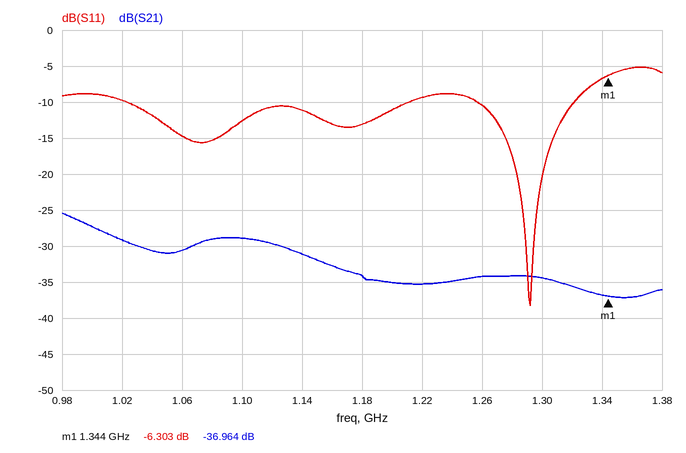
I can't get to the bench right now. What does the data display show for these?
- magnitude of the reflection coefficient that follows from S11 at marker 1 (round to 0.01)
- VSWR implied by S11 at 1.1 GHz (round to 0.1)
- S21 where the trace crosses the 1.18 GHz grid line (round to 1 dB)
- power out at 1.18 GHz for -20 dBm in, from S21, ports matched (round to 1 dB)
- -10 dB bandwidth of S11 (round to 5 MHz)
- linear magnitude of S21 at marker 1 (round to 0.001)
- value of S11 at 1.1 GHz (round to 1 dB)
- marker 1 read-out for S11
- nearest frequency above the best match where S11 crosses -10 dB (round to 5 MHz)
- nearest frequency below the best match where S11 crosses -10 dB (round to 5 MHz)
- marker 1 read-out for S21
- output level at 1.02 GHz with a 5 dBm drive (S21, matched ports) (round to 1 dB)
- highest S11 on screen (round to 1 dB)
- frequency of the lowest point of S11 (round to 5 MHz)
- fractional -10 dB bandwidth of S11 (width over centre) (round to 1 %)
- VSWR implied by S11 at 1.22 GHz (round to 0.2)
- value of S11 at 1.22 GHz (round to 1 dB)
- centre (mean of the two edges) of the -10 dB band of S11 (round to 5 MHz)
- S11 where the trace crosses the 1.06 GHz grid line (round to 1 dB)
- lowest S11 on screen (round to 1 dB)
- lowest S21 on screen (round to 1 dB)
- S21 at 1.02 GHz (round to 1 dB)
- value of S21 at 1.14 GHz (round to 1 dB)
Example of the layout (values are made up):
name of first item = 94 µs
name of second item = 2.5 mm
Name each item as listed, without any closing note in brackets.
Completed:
magnitude of the reflection coefficient that follows from S11 at marker 1 = 0.48
VSWR implied by S11 at 1.1 GHz = 1.6
S21 where the trace crosses the 1.18 GHz grid line = -34 dB
power out at 1.18 GHz for -20 dBm in, from S21, ports matched = -54 dBm
-10 dB bandwidth of S11 = 65 MHz
linear magnitude of S21 at marker 1 = 0.014
value of S11 at 1.1 GHz = -13 dB
marker 1 read-out for S11 = -6.303 dB
nearest frequency above the best match where S11 crosses -10 dB = 1.320 GHz
nearest frequency below the best match where S11 crosses -10 dB = 1.255 GHz
marker 1 read-out for S21 = -36.964 dB
output level at 1.02 GHz with a 5 dBm drive (S21, matched ports) = -24 dBm
highest S11 on screen = -5 dB
frequency of the lowest point of S11 = 1.290 GHz
fractional -10 dB bandwidth of S11 (width over centre) = 5 %
VSWR implied by S11 at 1.22 GHz = 2.0
value of S11 at 1.22 GHz = -9 dB
centre (mean of the two edges) of the -10 dB band of S11 = 1.290 GHz
S11 where the trace crosses the 1.06 GHz grid line = -15 dB
lowest S11 on screen = -38 dB
lowest S21 on screen = -37 dB
S21 at 1.02 GHz = -29 dB
value of S21 at 1.14 GHz = -31 dB
